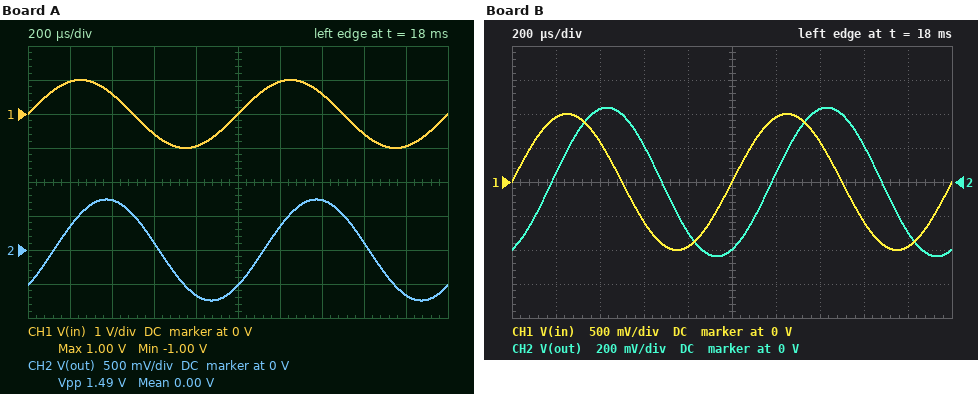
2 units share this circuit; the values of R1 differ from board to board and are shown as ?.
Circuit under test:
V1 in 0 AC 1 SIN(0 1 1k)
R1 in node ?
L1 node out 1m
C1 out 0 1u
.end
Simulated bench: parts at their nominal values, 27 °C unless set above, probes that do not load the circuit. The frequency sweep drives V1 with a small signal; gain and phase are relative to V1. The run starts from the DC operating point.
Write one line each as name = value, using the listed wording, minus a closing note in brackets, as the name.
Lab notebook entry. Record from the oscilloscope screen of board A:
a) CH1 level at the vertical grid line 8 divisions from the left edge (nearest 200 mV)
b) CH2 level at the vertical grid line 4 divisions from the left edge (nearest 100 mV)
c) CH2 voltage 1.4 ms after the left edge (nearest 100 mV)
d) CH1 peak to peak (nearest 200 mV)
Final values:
CH1 level at the vertical grid line 8 divisions from the left edge = -600 mV
CH2 level at the vertical grid line 4 divisions from the left edge = -700 mV
CH2 voltage 1.4 ms after the left edge = 700 mV
CH1 peak to peak = 2.0 V
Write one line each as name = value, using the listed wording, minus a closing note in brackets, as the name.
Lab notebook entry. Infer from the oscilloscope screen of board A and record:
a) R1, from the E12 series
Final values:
R1, from the E12 series = 150 Ω
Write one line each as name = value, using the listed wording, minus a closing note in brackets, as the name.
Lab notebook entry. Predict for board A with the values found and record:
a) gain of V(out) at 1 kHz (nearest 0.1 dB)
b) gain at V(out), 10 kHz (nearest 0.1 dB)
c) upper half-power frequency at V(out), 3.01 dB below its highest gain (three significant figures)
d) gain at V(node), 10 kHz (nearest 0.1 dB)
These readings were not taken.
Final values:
gain of V(out) at 1 kHz = -2.6 dB
gain at V(out), 10 kHz = -19.9 dB
upper half-power frequency at V(out), 3.01 dB below its highest gain = 1.11 kHz
gain at V(node), 10 kHz = -10.5 dB
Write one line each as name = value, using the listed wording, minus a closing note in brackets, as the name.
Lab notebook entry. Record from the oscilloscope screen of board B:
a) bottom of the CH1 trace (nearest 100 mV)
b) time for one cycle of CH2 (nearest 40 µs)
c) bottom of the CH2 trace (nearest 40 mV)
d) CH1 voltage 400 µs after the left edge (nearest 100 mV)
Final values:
bottom of the CH1 trace = -1.0 V
time for one cycle of CH2 = 1.00 ms
bottom of the CH2 trace = -440 mV
CH1 voltage 400 µs after the left edge = 600 mV
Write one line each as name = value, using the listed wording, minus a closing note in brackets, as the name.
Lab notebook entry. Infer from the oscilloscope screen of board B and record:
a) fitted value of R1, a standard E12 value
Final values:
fitted value of R1, a standard E12 value = 330 Ω
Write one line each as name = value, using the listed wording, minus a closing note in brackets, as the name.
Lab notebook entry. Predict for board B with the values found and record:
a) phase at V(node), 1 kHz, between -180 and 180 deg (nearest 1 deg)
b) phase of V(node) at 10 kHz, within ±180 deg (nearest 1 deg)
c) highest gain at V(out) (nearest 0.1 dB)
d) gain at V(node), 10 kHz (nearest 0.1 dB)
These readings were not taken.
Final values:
phase at V(node), 1 kHz, between -180 and 180 deg = -65 deg
phase of V(node) at 10 kHz, within ±180 deg = 82 deg
highest gain at V(out) = 0 dB
gain at V(node), 10 kHz = -17.0 dB
